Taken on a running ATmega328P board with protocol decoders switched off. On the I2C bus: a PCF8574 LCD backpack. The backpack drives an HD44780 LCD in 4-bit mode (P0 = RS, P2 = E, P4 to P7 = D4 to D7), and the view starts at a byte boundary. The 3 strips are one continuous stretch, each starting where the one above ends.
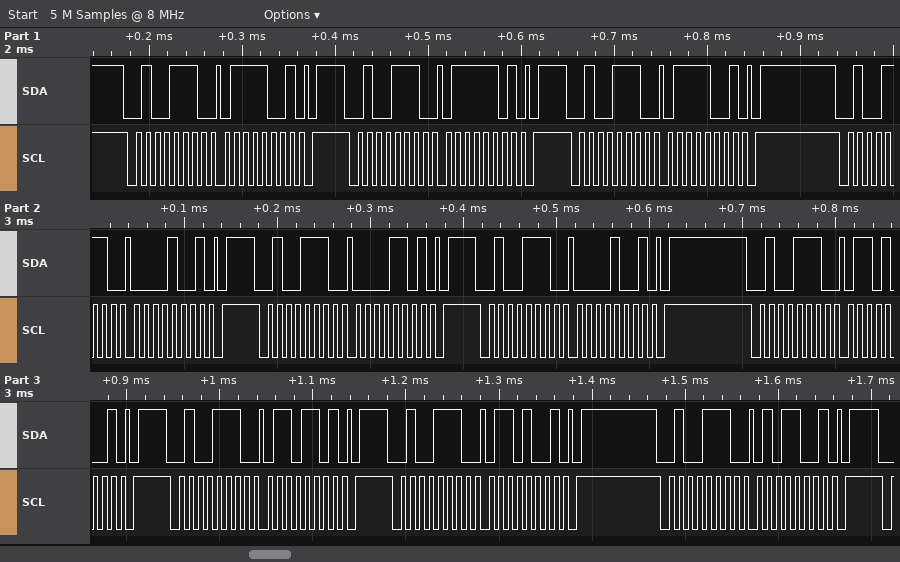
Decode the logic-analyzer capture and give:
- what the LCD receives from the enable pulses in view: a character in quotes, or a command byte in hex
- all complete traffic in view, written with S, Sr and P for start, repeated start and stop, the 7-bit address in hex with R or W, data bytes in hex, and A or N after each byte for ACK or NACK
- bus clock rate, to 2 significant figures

'p'
S 27W A 79 A P S 27W A 7D A P S 27W A 79 A P S 27W A 09 A P S 27W A 0D A P S 27W A 09 A P S 27W A 69 A P S 27W A 6D A P S 27W A 69 A P S 27W A 59 A P
100 kHz
